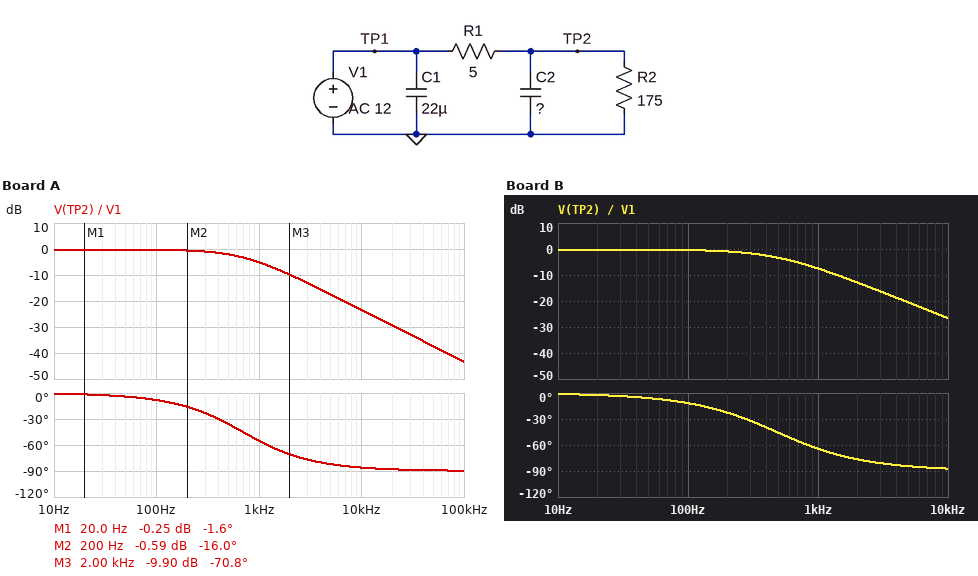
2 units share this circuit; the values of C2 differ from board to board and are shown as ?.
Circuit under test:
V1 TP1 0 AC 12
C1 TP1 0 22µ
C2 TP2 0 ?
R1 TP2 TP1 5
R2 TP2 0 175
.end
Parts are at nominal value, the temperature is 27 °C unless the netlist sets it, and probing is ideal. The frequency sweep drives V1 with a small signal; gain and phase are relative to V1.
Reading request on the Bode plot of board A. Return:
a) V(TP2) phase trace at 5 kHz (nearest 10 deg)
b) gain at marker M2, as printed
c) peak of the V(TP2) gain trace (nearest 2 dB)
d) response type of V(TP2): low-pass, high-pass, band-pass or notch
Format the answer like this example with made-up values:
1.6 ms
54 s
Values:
-80 deg
-0.59 dB
0 dB
low-pass
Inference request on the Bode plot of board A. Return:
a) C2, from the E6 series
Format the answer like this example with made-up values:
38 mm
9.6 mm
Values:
47 µF
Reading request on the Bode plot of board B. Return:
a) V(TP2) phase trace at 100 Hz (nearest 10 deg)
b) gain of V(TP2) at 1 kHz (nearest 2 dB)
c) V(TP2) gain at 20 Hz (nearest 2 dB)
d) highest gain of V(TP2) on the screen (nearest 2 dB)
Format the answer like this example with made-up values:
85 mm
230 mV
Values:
-10 deg
-8 dB
0 dB
0 dB
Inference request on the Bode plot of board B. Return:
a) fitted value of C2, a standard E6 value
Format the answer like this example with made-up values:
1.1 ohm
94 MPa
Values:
68 µF
